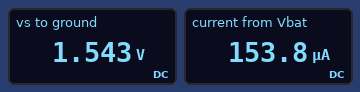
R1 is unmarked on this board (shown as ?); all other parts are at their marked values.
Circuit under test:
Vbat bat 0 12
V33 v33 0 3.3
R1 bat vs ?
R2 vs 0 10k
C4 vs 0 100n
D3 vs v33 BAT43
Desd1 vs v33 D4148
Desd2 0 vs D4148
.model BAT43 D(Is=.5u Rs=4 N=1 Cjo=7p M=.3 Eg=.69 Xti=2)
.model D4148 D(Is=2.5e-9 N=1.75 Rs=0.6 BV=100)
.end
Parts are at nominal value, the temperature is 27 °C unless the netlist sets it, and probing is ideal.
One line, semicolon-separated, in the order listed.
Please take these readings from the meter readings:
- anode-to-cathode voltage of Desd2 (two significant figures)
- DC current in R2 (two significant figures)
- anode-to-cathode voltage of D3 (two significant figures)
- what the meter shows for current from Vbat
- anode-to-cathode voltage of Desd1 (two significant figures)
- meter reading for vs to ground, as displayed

-1.5 V; 150 µA; -1.8 V; 153.8 µA; -1.8 V; 1.543 V
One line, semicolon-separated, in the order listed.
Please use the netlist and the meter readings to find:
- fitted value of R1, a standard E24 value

68 kΩ
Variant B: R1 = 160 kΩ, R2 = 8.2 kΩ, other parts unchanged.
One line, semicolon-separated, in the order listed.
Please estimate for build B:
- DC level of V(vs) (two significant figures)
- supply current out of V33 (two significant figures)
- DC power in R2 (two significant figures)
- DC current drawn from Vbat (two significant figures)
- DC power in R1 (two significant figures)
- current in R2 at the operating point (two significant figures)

590 mV; 500 nA; 42 µW; 71 µA; 810 µW; 72 µA
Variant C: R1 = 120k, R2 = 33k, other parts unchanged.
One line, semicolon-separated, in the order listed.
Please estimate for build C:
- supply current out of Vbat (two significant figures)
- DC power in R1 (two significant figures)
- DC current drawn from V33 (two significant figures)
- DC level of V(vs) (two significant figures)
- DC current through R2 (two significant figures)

78 µA; 740 µW; 500 nA; 2.6 V; 79 µA
